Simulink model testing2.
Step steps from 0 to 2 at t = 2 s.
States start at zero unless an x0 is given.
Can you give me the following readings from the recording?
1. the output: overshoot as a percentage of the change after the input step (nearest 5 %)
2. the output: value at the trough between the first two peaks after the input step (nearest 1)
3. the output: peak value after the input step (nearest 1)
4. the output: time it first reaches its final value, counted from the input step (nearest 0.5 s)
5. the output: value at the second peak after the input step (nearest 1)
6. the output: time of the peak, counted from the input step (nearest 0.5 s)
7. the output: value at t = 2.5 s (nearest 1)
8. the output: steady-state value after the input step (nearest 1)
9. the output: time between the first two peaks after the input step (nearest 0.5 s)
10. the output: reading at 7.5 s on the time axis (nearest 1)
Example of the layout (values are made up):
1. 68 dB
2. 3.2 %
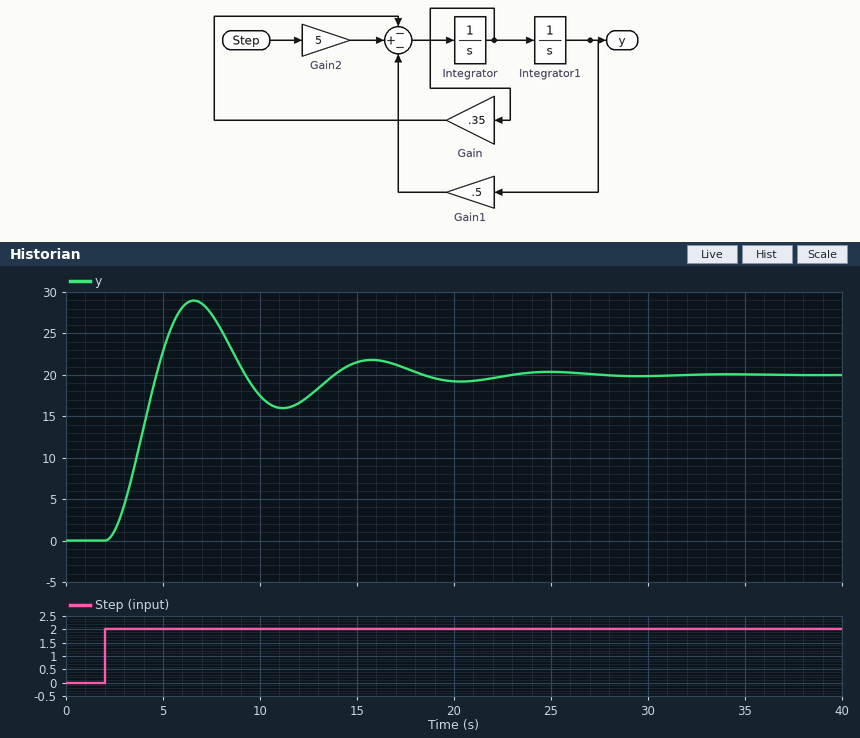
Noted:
1. 45 %
2. 16
3. 29
4. 2.5 s
5. 22
6. 4.5 s
7. 1
8. 20
9. 9.0 s
10. 27
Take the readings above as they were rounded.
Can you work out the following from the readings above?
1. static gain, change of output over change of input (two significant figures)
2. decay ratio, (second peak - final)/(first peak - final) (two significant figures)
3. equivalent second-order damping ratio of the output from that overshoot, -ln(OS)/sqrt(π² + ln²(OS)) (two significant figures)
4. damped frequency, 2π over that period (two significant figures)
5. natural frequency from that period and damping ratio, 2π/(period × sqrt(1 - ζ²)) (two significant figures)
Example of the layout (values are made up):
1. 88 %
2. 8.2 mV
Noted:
1. 10
2. 0.22
3. 0.25
4. 0.70 rad/s
5. 0.72 rad/s
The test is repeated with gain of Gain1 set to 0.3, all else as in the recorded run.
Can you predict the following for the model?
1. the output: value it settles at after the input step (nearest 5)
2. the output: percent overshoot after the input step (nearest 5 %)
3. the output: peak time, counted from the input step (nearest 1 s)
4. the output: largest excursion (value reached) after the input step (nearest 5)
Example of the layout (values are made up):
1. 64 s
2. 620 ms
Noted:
1. 35
2. 35 %
3. 6 s
4. 45
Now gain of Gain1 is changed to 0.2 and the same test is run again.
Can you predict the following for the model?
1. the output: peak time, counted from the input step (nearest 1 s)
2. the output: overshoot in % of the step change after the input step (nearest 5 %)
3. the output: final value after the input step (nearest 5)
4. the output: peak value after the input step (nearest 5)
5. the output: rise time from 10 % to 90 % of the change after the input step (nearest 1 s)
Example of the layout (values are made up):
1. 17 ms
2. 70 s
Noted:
1. 8 s
2. 25 %
3. 50
4. 65
5. 3 s
